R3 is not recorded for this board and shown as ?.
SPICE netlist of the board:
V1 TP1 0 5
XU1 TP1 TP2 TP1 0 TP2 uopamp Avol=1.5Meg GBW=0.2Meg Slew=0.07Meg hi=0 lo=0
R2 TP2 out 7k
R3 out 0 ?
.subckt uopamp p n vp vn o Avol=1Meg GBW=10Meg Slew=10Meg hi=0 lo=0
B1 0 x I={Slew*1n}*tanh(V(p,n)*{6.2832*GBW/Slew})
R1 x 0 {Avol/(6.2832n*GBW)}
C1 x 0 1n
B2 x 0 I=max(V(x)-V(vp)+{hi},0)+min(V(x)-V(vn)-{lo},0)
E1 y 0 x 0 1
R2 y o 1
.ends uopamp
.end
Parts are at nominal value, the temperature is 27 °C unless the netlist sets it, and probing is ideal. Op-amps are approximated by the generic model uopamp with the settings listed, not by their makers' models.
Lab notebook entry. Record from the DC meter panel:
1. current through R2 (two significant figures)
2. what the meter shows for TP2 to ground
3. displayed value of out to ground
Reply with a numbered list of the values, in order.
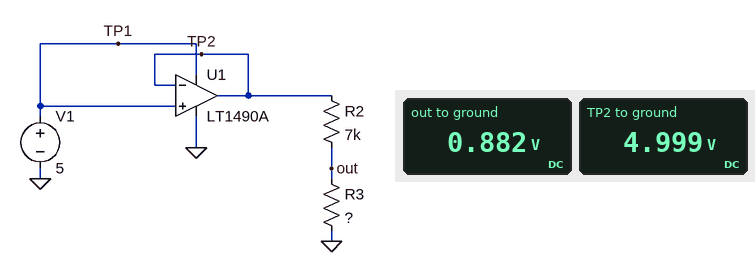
1. 590 µA
2. 4.999 V
3. 0.882 V
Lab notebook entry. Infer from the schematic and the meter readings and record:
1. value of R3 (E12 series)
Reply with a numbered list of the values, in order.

1. 1.5 kΩ
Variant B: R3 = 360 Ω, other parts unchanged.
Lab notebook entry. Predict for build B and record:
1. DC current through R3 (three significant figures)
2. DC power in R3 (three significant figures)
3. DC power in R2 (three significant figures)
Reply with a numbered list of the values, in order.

1. 679 µA
2. 166 µW
3. 3.23 mW
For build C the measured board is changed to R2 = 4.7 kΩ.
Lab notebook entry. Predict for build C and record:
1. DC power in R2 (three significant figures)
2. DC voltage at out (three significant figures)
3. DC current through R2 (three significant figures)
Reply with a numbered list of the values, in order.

1. 3.06 mW
2. 1.21 V
3. 806 µA
